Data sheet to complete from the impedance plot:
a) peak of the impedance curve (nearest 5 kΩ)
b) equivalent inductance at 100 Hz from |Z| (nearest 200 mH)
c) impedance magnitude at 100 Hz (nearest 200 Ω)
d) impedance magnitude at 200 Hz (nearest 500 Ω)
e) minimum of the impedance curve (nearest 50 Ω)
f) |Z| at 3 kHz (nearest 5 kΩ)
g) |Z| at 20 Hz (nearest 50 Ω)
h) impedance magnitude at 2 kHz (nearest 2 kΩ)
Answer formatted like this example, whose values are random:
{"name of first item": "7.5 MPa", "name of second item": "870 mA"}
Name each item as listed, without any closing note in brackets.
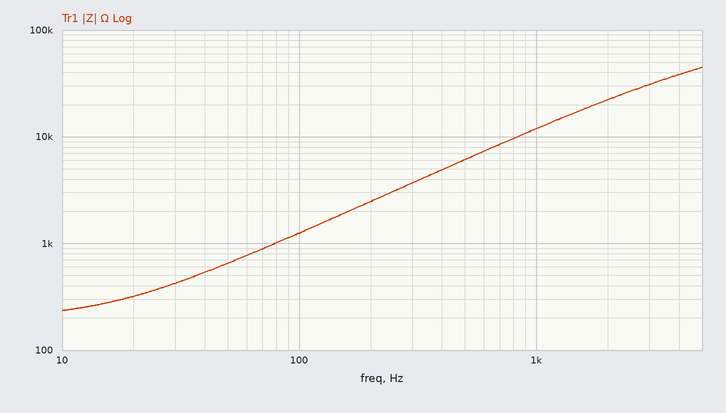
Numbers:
{"peak of the impedance curve": "45 kΩ", "equivalent inductance at 100 Hz from |Z|": "2.0 H", "impedance magnitude at 100 Hz": "1.2 kΩ", "impedance magnitude at 200 Hz": "2.5 kΩ", "minimum of the impedance curve": "250 Ω", "|Z| at 3 kHz": "30 kΩ", "|Z| at 20 Hz": "300 Ω", "impedance magnitude at 2 kHz": "22 kΩ"}
